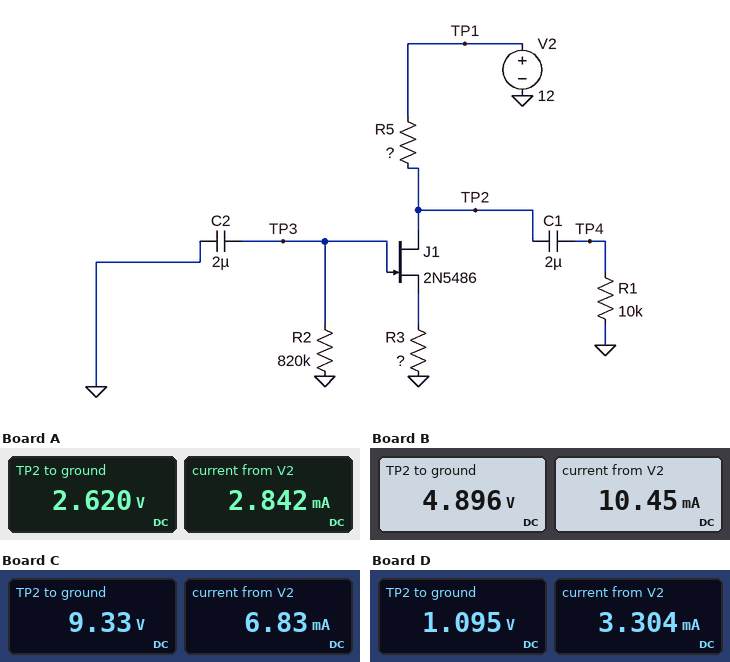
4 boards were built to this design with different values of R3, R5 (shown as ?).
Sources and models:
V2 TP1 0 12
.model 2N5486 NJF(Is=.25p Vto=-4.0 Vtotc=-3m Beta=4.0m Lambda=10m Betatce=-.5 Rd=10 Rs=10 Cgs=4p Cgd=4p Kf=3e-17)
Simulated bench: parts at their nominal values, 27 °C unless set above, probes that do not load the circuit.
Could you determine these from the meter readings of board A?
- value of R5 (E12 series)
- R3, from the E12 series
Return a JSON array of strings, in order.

["3.3 kΩ", "820 Ω"]
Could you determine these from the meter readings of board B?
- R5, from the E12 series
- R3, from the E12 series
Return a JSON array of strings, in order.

["680 Ω", "220 Ω"]
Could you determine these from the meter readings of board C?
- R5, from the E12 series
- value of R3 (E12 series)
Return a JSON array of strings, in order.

["390 Ω", "390 Ω"]
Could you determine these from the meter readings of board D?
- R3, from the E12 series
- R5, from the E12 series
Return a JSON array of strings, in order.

["270 Ω", "3.3 kΩ"]
